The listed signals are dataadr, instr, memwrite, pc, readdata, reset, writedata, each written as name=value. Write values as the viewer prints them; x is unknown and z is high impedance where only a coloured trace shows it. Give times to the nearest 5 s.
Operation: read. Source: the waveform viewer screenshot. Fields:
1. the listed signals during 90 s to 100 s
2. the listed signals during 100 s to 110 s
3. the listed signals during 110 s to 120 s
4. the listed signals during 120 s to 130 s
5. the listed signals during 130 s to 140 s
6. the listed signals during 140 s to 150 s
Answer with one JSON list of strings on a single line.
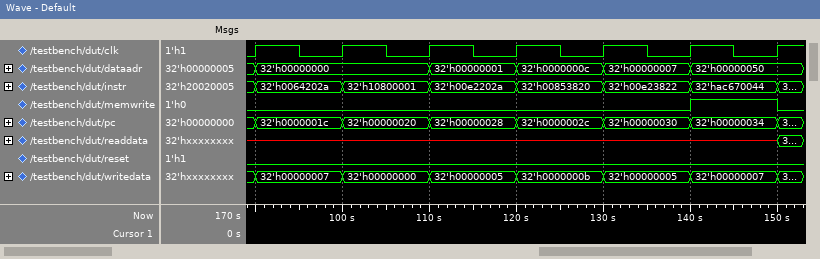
["dataadr=32'h00000000, instr=32'h0064202a, memwrite=0, pc=32'h0000001c, readdata=x, reset=0, writedata=32'h00000007", "dataadr=32'h00000000, instr=32'h10800001, memwrite=0, pc=32'h00000020, readdata=x, reset=0, writedata=32'h00000000", "dataadr=32'h00000001, instr=32'h00e2202a, memwrite=0, pc=32'h00000028, readdata=x, reset=0, writedata=32'h00000005", "dataadr=32'h0000000c, instr=32'h00853820, memwrite=0, pc=32'h0000002c, readdata=x, reset=0, writedata=32'h0000000b", "dataadr=32'h00000007, instr=32'h00e23822, memwrite=0, pc=32'h00000030, readdata=x, reset=0, writedata=32'h00000005", "dataadr=32'h00000050, instr=32'hac670044, memwrite=1, pc=32'h00000034, readdata=x, reset=0, writedata=32'h00000007"]
